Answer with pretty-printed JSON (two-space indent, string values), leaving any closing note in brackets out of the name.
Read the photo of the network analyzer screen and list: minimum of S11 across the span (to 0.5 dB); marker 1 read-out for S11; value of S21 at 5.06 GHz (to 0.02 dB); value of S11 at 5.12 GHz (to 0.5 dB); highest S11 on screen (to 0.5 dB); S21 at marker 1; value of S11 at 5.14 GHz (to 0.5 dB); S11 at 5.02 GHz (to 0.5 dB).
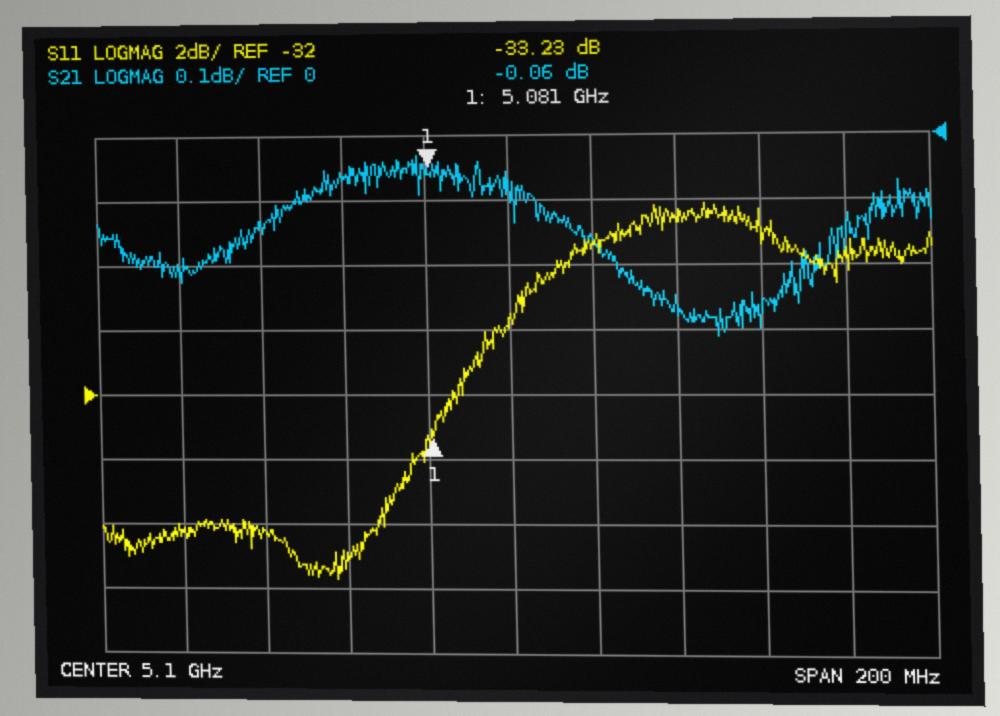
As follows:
{
  "minimum of S11 across the span": "-37.5 dB",
  "marker 1 read-out for S11": "-33.23 dB",
  "value of S21 at 5.06 GHz": "-0.06 dB",
  "value of S11 at 5.12 GHz": "-27.5 dB",
  "highest S11 on screen": "-26.0 dB",
  "S21 at marker 1": "-0.06 dB",
  "value of S11 at 5.14 GHz": "-26.5 dB",
  "S11 at 5.02 GHz": "-36.0 dB"
}
